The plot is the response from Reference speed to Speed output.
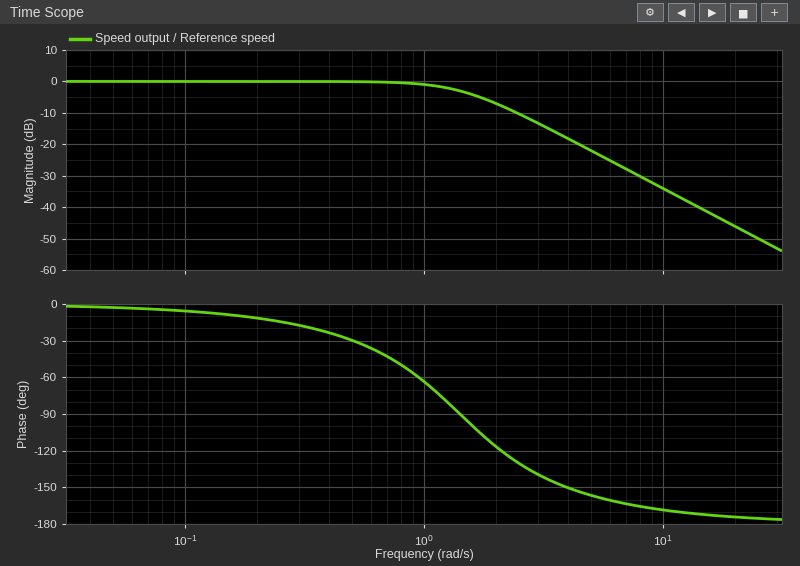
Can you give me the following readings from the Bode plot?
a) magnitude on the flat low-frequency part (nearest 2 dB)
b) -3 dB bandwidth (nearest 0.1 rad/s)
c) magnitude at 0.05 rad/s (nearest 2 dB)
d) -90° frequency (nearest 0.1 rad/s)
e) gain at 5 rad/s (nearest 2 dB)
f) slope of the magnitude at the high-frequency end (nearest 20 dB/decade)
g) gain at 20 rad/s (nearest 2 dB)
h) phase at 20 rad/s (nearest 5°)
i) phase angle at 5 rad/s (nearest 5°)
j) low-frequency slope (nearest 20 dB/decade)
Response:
0 dB
1.4 rad/s
0 dB
1.4 rad/s
-22 dB
-40 dB/decade
-46 dB
-175°
-155°
0 dB/decade
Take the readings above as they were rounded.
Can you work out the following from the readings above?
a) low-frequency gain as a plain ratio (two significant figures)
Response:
1.0
